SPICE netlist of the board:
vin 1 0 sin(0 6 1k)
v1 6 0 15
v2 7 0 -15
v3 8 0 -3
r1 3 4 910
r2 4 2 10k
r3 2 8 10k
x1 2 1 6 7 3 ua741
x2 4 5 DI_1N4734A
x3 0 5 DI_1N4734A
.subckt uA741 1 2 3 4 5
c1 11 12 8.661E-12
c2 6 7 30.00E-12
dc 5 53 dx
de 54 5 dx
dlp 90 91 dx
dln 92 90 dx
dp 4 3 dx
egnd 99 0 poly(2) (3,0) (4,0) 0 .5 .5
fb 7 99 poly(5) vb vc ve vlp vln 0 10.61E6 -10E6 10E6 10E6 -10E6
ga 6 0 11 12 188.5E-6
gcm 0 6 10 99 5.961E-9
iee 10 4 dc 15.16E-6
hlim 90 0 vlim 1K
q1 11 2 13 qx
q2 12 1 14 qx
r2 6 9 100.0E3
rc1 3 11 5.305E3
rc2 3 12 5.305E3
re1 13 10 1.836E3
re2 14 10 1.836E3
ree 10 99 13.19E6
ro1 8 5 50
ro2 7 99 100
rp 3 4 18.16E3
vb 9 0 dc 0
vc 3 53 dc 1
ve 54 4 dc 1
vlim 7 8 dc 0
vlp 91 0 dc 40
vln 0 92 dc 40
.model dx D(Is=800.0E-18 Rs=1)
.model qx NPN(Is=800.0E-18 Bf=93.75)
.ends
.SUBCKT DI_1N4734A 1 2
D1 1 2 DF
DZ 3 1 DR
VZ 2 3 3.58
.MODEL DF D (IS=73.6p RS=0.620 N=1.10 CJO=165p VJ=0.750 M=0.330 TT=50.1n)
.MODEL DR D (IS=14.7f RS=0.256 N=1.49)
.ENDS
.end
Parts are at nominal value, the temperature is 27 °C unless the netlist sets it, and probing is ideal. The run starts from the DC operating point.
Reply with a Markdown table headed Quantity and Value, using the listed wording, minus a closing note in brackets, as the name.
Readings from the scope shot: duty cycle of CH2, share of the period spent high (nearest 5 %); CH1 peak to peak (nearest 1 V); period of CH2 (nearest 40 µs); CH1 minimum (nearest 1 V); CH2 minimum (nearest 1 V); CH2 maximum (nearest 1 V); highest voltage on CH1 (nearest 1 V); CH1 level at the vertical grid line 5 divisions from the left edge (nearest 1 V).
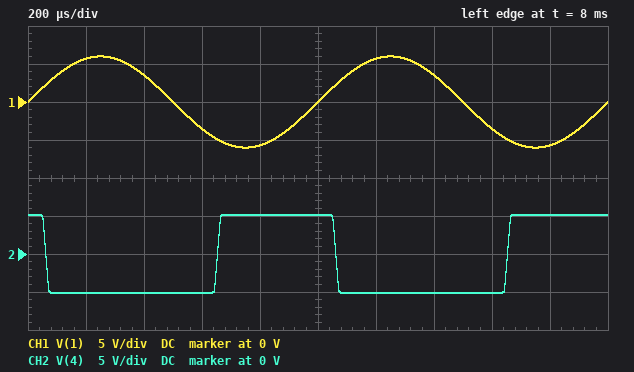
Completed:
| Quantity | Value |
|---|---|
| duty cycle of CH2, share of the period spent high | 40 % |
| CH1 peak to peak | 12 V |
| period of CH2 | 1.00 ms |
| CH1 minimum | -6 V |
| CH2 minimum | -5 V |
| CH2 maximum | 5 V |
| highest voltage on CH1 | 6 V |
| CH1 level at the vertical grid line 5 divisions from the left edge | 0 V |
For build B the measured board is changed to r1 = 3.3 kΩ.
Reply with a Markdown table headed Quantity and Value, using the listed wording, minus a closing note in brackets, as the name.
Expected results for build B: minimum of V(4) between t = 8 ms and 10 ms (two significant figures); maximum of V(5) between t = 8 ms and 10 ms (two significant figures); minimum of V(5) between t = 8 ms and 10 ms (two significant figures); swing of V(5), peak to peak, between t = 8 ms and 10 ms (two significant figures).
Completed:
| Quantity | Value |
|---|---|
| minimum of V(4) between t = 8 ms and 10 ms | -5.1 V |
| maximum of V(5) between t = 8 ms and 10 ms | 4.6 V |
| minimum of V(5) between t = 8 ms and 10 ms | -500 mV |
| swing of V(5), peak to peak, between t = 8 ms and 10 ms | 5.1 V |
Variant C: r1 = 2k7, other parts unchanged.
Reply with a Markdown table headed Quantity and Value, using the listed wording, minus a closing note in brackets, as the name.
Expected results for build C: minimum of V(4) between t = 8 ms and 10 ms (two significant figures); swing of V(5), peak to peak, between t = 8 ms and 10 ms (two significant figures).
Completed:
| Quantity | Value |
|---|---|
| minimum of V(4) between t = 8 ms and 10 ms | -5.1 V |
| swing of V(5), peak to peak, between t = 8 ms and 10 ms | 5.1 V |
